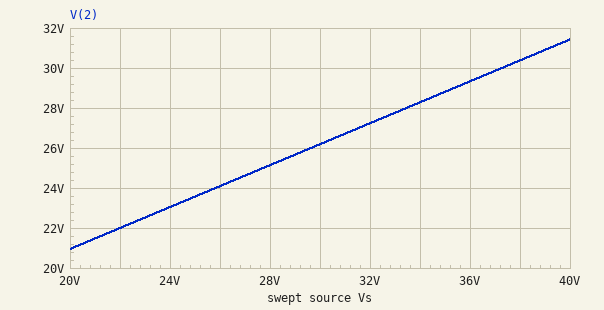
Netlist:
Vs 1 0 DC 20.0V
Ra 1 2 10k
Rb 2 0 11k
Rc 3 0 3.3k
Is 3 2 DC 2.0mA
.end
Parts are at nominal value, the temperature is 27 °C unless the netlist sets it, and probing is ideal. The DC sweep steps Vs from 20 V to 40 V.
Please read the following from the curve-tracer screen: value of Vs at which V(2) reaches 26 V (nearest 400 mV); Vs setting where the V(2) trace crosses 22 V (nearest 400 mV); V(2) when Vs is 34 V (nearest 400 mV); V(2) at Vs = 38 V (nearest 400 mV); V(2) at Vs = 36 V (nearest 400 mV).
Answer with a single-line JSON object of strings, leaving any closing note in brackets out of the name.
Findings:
{"value of Vs at which V(2) reaches 26 V": "29.6 V", "Vs setting where the V(2) trace crosses 22 V": "22.0 V", "V(2) when Vs is 34 V": "28.4 V", "V(2) at Vs = 38 V": "30.4 V", "V(2) at Vs = 36 V": "29.2 V"}
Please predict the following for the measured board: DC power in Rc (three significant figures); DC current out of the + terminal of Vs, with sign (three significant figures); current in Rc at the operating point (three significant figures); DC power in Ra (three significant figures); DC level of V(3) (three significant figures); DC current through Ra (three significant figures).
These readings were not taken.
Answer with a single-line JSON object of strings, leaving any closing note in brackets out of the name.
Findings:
{"DC power in Rc": "13.2 mW", "DC current out of the + terminal of Vs, with sign": "-95.2 µA", "current in Rc at the operating point": "2.00 mA", "DC power in Ra": "90.7 µW", "DC level of V(3)": "-6.60 V", "DC current through Ra": "95.2 µA"}
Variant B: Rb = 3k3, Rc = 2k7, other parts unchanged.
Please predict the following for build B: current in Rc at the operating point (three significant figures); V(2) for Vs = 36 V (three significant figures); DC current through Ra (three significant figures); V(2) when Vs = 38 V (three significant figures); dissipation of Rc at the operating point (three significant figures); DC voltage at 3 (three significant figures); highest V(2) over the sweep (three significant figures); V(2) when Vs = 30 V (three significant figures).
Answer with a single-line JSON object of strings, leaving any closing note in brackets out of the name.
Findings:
{"current in Rc at the operating point": "2.00 mA", "V(2) for Vs = 36 V": "13.9 V", "DC current through Ra": "1.01 mA", "V(2) when Vs = 38 V": "14.4 V", "dissipation of Rc at the operating point": "10.8 mW", "DC voltage at 3": "-5.40 V", "highest V(2) over the sweep": "14.9 V", "V(2) when Vs = 30 V": "12.4 V"}
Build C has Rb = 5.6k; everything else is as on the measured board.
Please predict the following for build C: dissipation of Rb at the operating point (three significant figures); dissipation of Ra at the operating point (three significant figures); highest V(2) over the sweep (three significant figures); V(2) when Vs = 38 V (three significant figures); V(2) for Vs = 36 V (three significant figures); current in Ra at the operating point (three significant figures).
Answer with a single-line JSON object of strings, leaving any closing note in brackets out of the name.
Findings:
{"dissipation of Rb at the operating point": "36.8 mW", "dissipation of Ra at the operating point": "3.18 mW", "highest V(2) over the sweep": "21.5 V", "V(2) when Vs = 38 V": "20.8 V", "V(2) for Vs = 36 V": "20.1 V", "current in Ra at the operating point": "564 µA"}
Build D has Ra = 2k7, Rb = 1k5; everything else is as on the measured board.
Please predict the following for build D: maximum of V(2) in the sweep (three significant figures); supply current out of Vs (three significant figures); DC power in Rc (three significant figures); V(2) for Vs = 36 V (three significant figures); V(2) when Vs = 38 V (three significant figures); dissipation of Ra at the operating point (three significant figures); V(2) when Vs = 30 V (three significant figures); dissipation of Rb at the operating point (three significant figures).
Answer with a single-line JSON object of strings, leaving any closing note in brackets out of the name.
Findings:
{"maximum of V(2) in the sweep": "16.2 V", "supply current out of Vs": "4.05 mA", "DC power in Rc": "13.2 mW", "V(2) for Vs = 36 V": "14.8 V", "V(2) when Vs = 38 V": "15.5 V", "dissipation of Ra at the operating point": "44.2 mW", "V(2) when Vs = 30 V": "12.6 V", "dissipation of Rb at the operating point": "54.9 mW"}
